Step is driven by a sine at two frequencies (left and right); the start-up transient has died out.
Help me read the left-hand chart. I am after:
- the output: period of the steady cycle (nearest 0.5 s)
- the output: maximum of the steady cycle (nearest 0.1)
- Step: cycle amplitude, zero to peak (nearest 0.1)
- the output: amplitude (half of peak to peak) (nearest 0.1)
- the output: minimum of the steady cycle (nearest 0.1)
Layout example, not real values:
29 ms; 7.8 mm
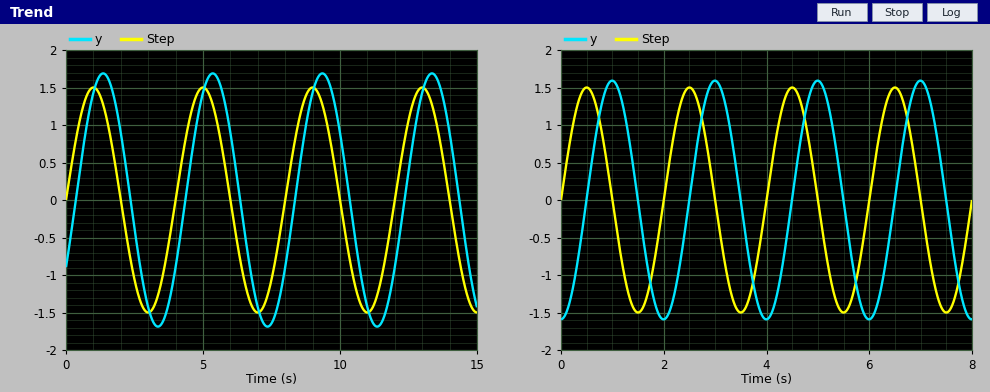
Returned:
4.0 s; 1.7; 1.5; 1.7; -1.7
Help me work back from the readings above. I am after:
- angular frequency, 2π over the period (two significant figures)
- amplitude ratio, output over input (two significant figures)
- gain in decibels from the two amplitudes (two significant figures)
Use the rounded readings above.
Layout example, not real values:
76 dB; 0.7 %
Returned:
1.6 rad/s; 1.1; 1.1 dB
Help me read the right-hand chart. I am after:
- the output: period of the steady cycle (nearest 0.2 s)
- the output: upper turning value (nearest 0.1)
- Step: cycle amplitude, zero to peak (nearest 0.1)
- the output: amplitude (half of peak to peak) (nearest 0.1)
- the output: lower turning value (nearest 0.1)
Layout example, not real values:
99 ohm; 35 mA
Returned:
2.0 s; 1.6; 1.5; 1.6; -1.6
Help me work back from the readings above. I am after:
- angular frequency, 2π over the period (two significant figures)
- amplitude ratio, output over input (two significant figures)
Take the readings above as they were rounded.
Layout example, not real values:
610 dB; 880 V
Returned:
3.1 rad/s; 1.1
